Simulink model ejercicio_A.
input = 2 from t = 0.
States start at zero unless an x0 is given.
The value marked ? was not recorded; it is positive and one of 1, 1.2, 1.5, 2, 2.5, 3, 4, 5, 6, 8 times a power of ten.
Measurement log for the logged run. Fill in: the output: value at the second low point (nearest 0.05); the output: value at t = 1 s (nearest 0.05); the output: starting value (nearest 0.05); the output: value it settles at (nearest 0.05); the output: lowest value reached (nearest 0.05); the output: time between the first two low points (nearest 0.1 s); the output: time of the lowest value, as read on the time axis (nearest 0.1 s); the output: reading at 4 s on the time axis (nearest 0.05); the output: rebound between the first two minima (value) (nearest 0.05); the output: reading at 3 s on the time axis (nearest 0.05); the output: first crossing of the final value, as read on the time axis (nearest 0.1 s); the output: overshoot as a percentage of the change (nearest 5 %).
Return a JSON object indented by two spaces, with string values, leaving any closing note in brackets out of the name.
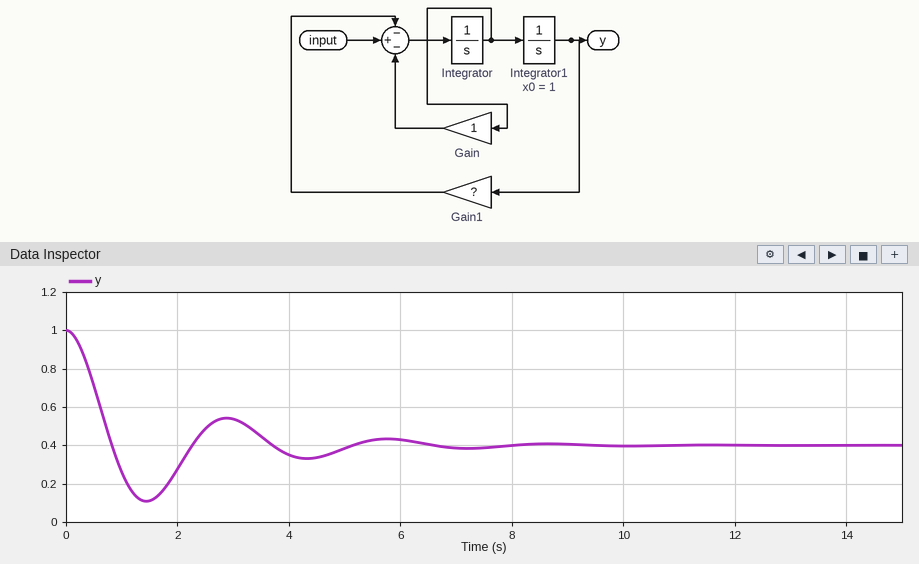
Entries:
{
  "the output: value at the second low point": "0.35",
  "the output: value at t = 1 s": "0.25",
  "the output: starting value": "1.00",
  "the output: value it settles at": "0.40",
  "the output: lowest value reached": "0.10",
  "the output: time between the first two low points": "2.9 s",
  "the output: time of the lowest value, as read on the time axis": "1.4 s",
  "the output: reading at 4 s on the time axis": "0.35",
  "the output: rebound between the first two minima (value)": "0.55",
  "the output: reading at 3 s on the time axis": "0.55",
  "the output: first crossing of the final value, as read on the time axis": "0.8 s",
  "the output: overshoot as a percentage of the change": "50 %"
}
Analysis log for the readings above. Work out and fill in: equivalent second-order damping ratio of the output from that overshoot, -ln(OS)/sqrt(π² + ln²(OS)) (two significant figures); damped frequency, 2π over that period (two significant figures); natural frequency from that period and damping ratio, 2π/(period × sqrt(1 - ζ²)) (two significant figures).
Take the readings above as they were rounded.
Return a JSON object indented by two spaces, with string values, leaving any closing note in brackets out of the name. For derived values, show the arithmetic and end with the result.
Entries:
{
  "equivalent second-order damping ratio of the output from that overshoot, -ln(OS)/sqrt(π² + ln²(OS))": "ln(0.5) = -0.693; 0.693 / sqrt(9.870 + 0.480) = 0.22",
  "damped frequency, 2π over that period": "2π / 2.9 = 2.2 rad/s",
  "natural frequency from that period and damping ratio, 2π/(period × sqrt(1 - ζ²))": "2π / (2.9 × sqrt(1 - 0.22²)) = 2.2 rad/s"
}
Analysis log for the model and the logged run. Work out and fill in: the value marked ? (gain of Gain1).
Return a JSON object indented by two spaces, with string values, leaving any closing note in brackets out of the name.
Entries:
{
  "the value marked ?": "5"
}
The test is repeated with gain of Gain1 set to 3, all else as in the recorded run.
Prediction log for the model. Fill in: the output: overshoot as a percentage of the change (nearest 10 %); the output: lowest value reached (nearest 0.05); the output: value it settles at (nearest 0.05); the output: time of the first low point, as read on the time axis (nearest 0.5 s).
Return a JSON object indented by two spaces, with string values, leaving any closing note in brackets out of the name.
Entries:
{
  "the output: overshoot as a percentage of the change": "40 %",
  "the output: lowest value reached": "0.55",
  "the output: value it settles at": "0.65",
  "the output: time of the first low point, as read on the time axis": "2.0 s"
}
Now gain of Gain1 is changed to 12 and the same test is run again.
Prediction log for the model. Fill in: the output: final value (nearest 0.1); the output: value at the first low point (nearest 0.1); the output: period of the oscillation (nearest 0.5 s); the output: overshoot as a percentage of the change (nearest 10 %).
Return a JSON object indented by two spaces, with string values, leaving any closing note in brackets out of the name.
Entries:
{
  "the output: final value": "0.2",
  "the output: value at the first low point": "-0.4",
  "the output: period of the oscillation": "2.0 s",
  "the output: overshoot as a percentage of the change": "60 %"
}
